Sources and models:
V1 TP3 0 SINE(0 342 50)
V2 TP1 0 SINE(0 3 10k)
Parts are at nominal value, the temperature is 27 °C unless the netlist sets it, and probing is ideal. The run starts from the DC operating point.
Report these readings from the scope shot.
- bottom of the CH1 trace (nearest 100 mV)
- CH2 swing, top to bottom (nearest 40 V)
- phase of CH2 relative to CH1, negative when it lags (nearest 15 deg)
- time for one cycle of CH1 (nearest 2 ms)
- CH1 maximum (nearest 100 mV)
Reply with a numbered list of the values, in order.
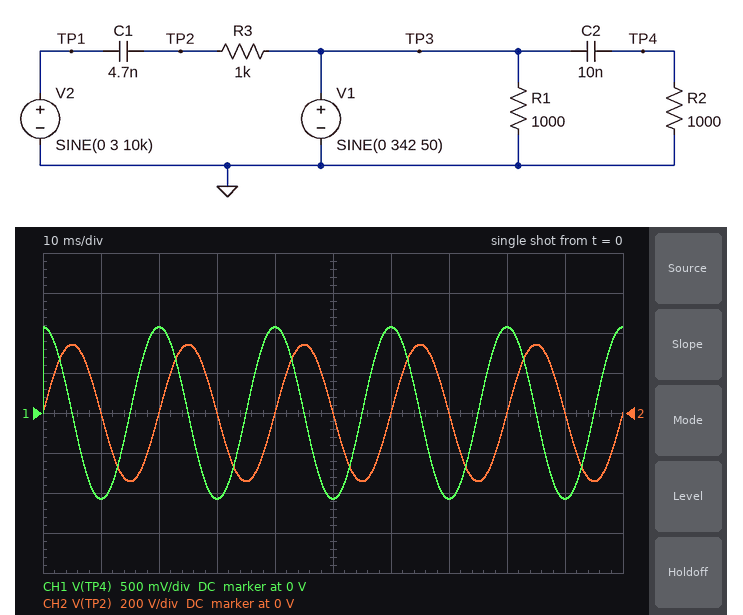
1. -1.1 V
2. 680 V
3. -90 deg
4. 20 ms
5. 1.1 V
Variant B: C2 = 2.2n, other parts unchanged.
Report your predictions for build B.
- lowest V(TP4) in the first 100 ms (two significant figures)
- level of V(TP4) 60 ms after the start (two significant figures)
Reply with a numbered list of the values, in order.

1. -240 mV
2. 240 mV
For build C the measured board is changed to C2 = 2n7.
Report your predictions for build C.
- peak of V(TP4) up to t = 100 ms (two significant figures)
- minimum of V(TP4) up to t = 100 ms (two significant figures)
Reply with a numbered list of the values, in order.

1. 290 mV
2. -290 mV
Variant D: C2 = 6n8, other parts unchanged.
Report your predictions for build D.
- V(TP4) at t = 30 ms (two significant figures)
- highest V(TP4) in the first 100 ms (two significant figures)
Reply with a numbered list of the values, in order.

1. -730 mV
2. 730 mV
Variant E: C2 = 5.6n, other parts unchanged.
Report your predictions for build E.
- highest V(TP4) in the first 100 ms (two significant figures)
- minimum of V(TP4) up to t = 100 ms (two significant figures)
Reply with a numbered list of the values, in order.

1. 600 mV
2. -600 mV
